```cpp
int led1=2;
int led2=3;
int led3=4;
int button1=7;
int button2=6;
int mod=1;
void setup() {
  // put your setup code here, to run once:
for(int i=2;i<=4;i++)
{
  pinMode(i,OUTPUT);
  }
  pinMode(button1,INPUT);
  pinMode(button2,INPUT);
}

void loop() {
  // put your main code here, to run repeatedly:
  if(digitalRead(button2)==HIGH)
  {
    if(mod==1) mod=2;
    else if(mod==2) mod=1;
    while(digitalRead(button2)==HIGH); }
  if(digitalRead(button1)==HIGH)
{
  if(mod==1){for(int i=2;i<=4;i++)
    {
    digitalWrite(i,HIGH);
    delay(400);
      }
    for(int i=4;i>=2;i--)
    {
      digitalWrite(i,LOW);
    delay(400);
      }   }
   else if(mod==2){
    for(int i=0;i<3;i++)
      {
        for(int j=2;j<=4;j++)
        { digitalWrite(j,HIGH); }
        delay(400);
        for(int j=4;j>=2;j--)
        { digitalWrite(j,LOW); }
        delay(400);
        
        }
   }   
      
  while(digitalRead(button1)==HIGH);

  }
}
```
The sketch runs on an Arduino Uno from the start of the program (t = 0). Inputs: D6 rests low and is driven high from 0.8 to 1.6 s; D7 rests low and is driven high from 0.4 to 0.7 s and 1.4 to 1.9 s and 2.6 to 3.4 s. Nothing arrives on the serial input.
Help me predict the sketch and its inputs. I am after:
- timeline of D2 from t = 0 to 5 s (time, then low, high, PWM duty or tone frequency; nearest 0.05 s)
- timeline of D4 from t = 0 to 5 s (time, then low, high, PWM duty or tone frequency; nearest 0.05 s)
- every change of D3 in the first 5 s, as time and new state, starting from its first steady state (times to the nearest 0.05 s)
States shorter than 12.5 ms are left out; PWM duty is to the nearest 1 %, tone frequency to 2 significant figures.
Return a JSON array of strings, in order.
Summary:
["0 s low; 0.4 s high; 2.4 s low", "0 s low; 1.2 s high; 1.6 s low", "0 s low; 0.8 s high; 2 s low"]
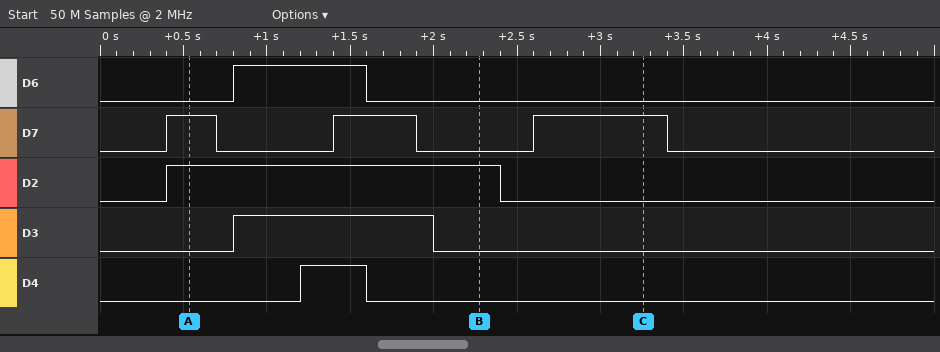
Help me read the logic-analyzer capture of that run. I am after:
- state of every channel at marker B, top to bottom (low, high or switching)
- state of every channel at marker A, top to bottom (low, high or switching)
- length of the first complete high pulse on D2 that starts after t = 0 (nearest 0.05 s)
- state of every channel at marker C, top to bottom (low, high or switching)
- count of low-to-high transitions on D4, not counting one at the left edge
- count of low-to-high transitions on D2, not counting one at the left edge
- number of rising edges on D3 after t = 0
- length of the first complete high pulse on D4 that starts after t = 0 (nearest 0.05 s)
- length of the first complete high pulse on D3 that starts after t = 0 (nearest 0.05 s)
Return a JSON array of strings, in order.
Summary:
["D6 low, D7 low, D2 high, D3 low, D4 low", "D6 low, D7 high, D2 high, D3 low, D4 low", "2.00 s", "D6 low, D7 high, D2 low, D3 low, D4 low", "1", "1", "1", "0.40 s", "1.20 s"]
